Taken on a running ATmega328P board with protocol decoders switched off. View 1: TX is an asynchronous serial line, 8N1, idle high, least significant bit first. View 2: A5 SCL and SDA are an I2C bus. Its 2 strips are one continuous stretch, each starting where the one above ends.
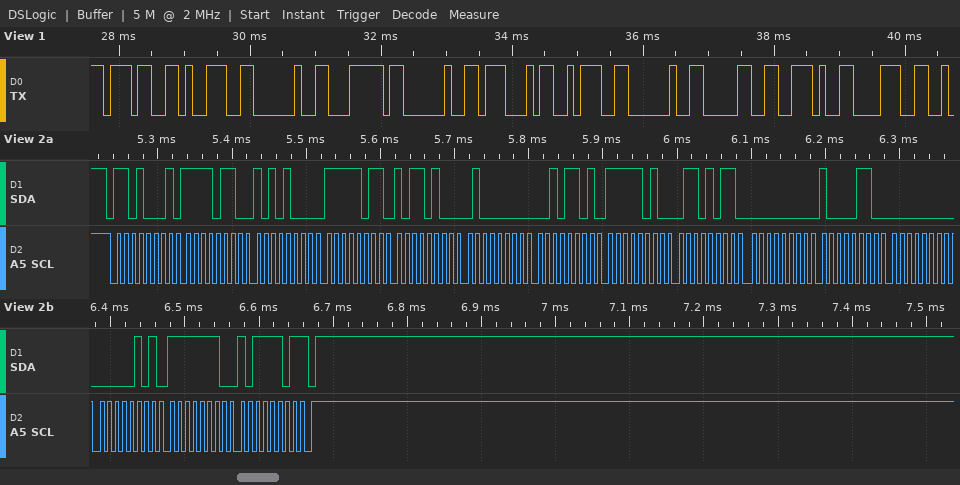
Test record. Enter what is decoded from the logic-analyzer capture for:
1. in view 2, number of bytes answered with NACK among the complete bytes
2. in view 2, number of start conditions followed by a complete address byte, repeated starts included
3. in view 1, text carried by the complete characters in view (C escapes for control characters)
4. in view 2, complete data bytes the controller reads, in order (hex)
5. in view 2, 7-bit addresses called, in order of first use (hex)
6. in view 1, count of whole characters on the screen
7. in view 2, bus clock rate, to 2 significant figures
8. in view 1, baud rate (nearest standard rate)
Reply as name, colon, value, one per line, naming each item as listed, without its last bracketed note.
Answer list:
in view 2, number of bytes answered with NACK among the complete bytes: 1
in view 2, number of start conditions followed by a complete address byte, repeated starts included: 1
in view 1, text carried by the complete characters in view: "79 | G: 0.8"
in view 2, complete data bytes the controller reads, in order: F6 A8 FB B4 40 2D FA 6B 00 86 00 05 FE BD
in view 2, 7-bit addresses called, in order of first use: 0x68
in view 1, count of whole characters on the screen: 11
in view 2, bus clock rate, to 2 significant figures: 100 kHz
in view 1, baud rate: 9600 baud
